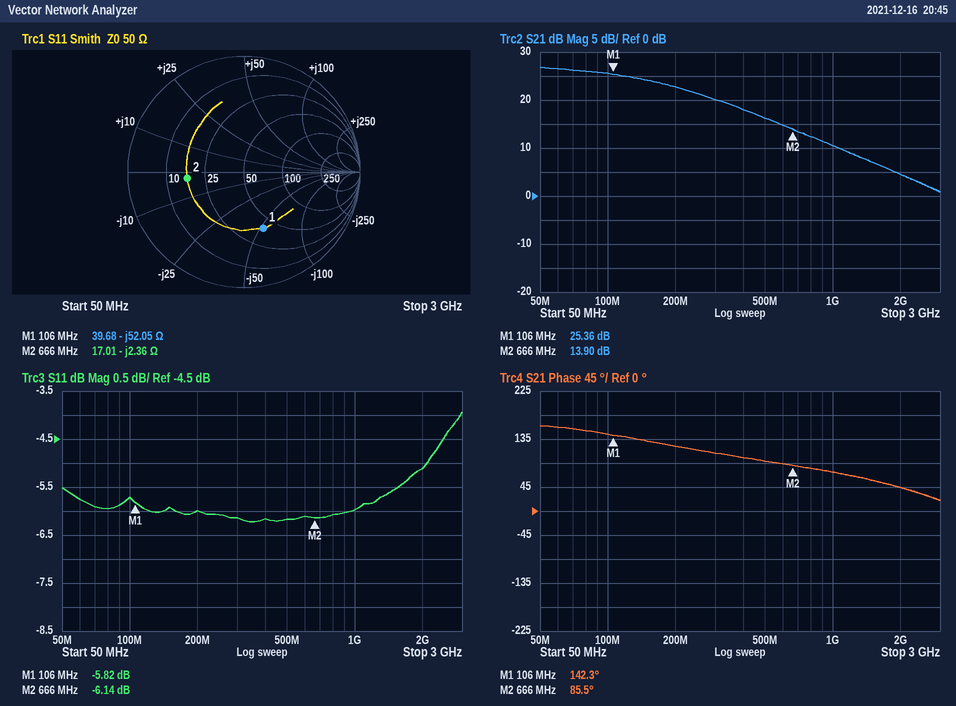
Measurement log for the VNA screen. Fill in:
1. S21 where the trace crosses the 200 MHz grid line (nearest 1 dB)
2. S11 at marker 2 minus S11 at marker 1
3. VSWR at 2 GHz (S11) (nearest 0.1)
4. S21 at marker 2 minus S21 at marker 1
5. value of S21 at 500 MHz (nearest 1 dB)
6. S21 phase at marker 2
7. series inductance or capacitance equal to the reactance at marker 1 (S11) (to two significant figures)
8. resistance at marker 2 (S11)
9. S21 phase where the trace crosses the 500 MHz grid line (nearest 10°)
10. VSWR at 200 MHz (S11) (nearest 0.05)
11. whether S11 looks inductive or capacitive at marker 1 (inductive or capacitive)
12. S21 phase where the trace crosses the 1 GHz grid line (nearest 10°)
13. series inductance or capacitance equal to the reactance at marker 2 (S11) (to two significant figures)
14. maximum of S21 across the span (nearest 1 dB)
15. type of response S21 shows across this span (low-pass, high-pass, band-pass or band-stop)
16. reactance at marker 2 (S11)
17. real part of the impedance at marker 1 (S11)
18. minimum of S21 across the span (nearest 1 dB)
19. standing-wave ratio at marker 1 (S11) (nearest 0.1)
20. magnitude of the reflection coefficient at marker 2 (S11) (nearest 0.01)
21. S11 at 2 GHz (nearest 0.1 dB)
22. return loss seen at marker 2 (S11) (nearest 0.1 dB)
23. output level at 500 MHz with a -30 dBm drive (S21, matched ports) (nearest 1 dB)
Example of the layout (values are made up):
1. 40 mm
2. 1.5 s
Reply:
1. 23 dB
2. -0.32 dB
3. 3.5
4. -11.46 dB
5. 16 dB
6. 85.5°
7. 29 pF
8. 17.01 Ω
9. 90°
10. 3.00
11. capacitive
12. 70°
13. 100 pF
14. 27 dB
15. low-pass
16. -2.36 Ω
17. 39.68 Ω
18. 1 dB
19. 3.1
20. 0.49
21. -5.1 dB
22. 6.1 dB
23. -14 dBm
